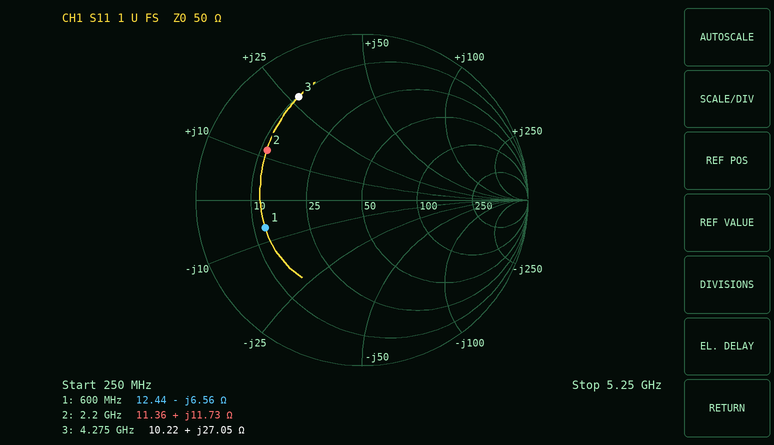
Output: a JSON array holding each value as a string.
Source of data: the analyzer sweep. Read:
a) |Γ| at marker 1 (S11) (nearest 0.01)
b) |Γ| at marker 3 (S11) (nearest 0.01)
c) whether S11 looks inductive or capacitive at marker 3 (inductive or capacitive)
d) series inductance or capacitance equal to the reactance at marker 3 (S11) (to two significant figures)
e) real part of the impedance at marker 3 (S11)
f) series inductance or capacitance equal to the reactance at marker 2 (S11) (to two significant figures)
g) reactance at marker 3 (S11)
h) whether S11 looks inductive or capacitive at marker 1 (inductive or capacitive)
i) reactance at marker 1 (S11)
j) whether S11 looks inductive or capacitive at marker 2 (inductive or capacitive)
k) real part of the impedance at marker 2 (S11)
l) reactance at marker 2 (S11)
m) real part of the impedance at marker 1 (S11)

["0.61", "0.73", "inductive", "1.0 nH", "10.22 Ω", "850 pH", "+27.05 Ω", "capacitive", "-6.56 Ω", "inductive", "11.36 Ω", "+11.73 Ω", "12.44 Ω"]
